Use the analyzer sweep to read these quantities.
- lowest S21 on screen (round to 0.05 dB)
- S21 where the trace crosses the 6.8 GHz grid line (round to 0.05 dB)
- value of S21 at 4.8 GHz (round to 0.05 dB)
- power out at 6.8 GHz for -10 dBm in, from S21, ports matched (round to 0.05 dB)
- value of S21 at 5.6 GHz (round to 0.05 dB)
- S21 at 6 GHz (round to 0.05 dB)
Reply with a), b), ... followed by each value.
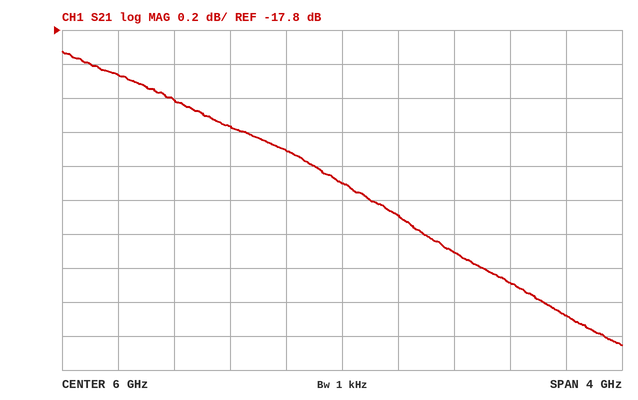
a) -19.65 dB
b) -19.10 dB
c) -18.20 dB
d) -29.10 dBm
e) -18.50 dB
f) -18.70 dB
